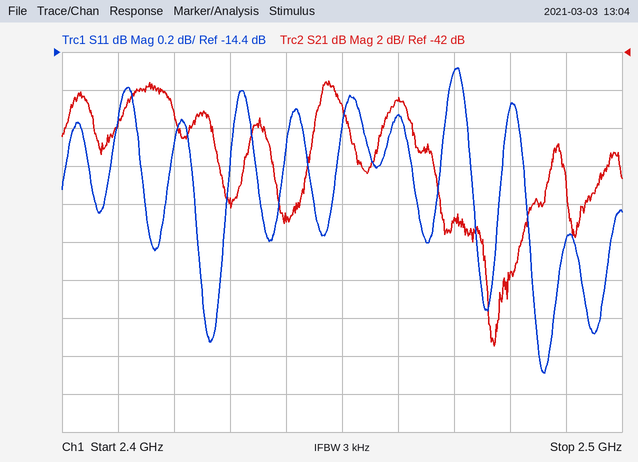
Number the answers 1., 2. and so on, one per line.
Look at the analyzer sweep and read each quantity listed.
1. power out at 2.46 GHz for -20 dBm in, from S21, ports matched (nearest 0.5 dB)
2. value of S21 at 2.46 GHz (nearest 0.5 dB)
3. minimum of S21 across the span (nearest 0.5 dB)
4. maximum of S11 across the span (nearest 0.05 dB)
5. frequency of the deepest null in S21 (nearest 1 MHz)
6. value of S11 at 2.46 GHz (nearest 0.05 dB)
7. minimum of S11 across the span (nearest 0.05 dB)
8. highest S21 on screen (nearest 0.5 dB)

1. -64.5 dBm
2. -44.5 dB
3. -57.5 dB
4. -14.50 dB
5. 2.477 GHz
6. -14.75 dB
7. -16.10 dB
8. -43.5 dB
